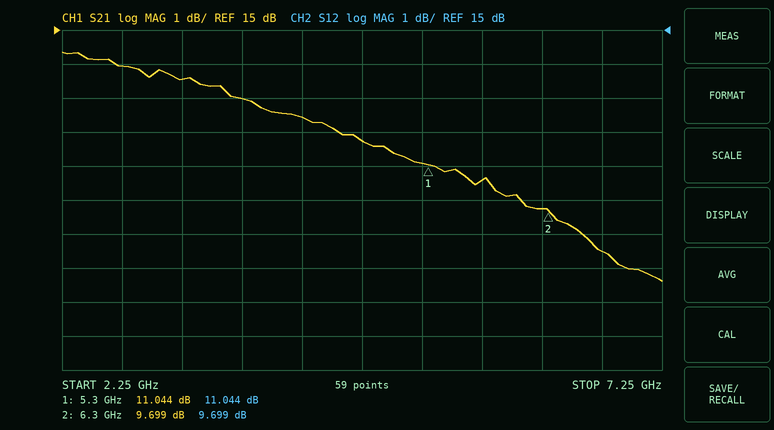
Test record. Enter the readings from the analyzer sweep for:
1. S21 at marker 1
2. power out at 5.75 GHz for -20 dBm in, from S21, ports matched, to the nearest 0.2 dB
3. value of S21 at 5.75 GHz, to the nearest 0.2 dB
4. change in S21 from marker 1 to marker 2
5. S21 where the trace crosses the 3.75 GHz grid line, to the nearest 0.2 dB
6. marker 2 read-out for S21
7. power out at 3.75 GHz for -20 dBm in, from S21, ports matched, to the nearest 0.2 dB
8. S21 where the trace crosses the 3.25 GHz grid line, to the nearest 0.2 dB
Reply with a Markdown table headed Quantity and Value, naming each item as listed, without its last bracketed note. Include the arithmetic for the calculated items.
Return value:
| Quantity | Value |
|---|---|
| S21 at marker 1 | 11.044 dB |
| power out at 5.75 GHz for -20 dBm in, from S21, ports matched, to the nearest 0.2 dB | -20 dBm + (10.6 dB) = -9.4 dBm |
| value of S21 at 5.75 GHz, to the nearest 0.2 dB | 10.6 dB |
| change in S21 from marker 1 to marker 2 | 9.699 − (11.044) = -1.345 dB |
| S21 where the trace crosses the 3.75 GHz grid line, to the nearest 0.2 dB | 13.0 dB |
| marker 2 read-out for S21 | 9.699 dB |
| power out at 3.75 GHz for -20 dBm in, from S21, ports matched, to the nearest 0.2 dB | -20 dBm + (13.0 dB) = -7.0 dBm |
| S21 where the trace crosses the 3.25 GHz grid line, to the nearest 0.2 dB | 13.6 dB |
